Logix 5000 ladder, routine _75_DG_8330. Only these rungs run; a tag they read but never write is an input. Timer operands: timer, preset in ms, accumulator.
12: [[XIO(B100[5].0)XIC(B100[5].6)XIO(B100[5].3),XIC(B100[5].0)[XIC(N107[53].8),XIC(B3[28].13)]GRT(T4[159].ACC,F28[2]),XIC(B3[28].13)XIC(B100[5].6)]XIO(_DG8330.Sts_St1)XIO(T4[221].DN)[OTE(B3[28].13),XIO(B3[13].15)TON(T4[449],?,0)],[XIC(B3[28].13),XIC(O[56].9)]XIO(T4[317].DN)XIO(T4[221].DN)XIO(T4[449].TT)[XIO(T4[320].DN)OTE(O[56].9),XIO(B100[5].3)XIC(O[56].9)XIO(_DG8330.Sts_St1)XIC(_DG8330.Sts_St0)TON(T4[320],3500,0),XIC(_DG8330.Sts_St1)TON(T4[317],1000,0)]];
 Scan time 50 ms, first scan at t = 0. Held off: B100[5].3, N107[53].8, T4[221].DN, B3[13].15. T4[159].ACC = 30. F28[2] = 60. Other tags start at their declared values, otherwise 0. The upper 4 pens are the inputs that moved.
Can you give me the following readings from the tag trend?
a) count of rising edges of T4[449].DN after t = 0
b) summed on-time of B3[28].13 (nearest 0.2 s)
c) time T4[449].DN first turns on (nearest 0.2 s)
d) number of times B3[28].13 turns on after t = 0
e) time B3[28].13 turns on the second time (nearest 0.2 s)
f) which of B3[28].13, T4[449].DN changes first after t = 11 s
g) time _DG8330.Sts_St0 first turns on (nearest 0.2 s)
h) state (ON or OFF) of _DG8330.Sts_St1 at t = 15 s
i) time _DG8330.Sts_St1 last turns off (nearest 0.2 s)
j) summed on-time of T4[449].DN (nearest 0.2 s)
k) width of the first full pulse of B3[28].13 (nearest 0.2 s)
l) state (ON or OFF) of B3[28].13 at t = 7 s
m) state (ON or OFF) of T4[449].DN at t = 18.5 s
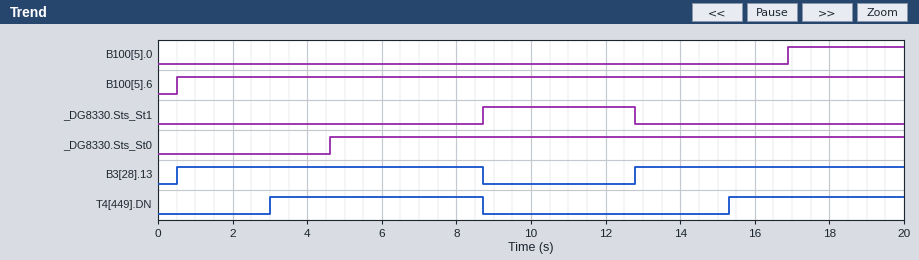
2
15.4 s
3.0 s
2
12.8 s
B3[28].13
4.6 s
OFF
12.8 s
10.4 s
8.2 s
ON
ON
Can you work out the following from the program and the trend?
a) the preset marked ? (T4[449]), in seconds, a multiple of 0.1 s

2.5 s
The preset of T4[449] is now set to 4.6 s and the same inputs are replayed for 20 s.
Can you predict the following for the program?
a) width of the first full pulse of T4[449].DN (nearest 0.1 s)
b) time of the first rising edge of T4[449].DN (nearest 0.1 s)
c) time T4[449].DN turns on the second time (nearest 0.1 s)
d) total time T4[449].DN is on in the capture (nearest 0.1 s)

3.6 s
5.1 s
17.4 s
6.2 s
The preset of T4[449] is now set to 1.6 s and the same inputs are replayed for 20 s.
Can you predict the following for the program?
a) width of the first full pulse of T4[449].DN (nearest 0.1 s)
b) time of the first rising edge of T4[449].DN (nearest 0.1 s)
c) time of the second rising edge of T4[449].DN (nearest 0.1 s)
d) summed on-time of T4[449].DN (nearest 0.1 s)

6.6 s
2.1 s
14.4 s
12.2 s
